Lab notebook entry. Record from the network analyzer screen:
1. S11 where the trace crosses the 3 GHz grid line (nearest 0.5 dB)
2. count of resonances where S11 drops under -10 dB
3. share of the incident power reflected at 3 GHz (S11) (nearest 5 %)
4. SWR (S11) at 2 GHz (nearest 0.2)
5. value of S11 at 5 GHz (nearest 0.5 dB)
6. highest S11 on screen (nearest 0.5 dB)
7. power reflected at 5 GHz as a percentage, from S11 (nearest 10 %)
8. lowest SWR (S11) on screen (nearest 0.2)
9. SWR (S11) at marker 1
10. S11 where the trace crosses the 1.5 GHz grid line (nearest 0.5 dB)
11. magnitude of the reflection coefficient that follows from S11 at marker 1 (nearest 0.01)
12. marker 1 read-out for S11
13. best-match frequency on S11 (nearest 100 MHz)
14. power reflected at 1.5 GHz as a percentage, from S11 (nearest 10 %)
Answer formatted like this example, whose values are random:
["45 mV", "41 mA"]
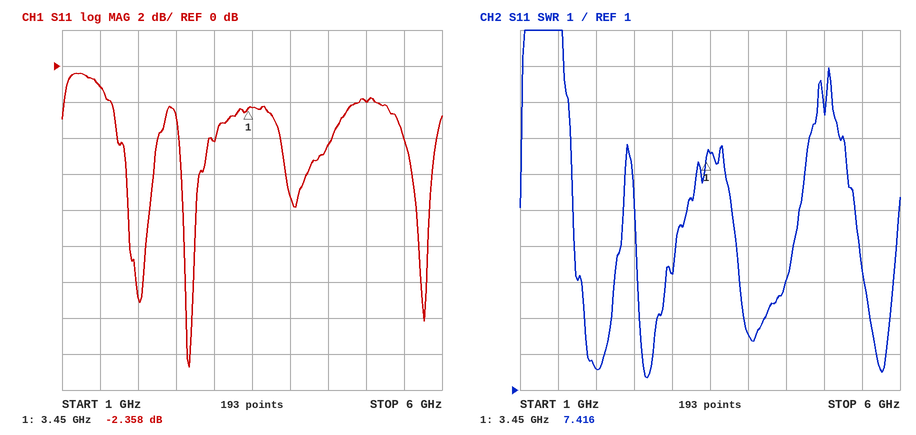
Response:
["-4.0 dB", "3", "40 %", "1.6", "-2.0 dB", "-0.5 dB", "60 %", "1.4", "7.416", "-1.0 dB", "0.76", "-2.358 dB", "2.7 GHz", "80 %"]
